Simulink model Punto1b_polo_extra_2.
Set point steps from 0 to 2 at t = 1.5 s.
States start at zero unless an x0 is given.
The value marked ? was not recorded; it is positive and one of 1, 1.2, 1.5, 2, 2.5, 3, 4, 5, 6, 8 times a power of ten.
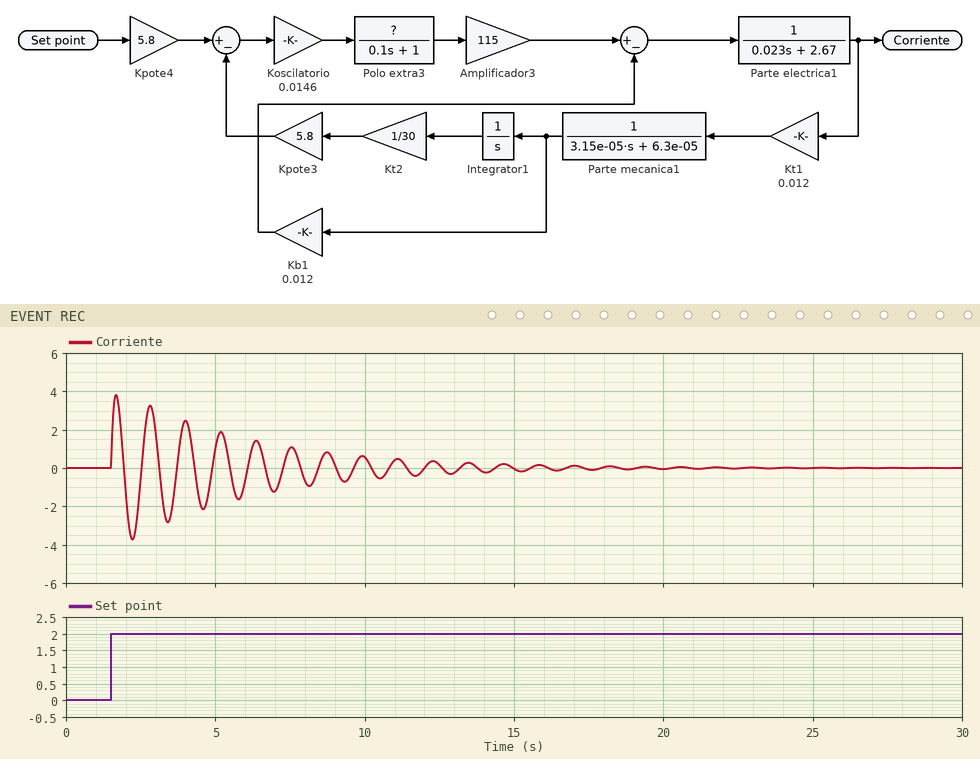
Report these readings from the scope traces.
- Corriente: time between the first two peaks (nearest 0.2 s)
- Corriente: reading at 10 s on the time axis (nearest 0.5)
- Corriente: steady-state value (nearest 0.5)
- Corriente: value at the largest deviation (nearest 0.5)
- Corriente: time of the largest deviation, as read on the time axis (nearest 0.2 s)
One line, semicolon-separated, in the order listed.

1.2 s; 0.5; 0.0; 4.0; 1.6 s
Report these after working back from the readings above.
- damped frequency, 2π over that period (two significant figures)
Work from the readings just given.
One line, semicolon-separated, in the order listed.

5.2 rad/s
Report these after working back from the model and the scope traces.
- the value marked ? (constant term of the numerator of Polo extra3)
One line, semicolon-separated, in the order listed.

0.8
